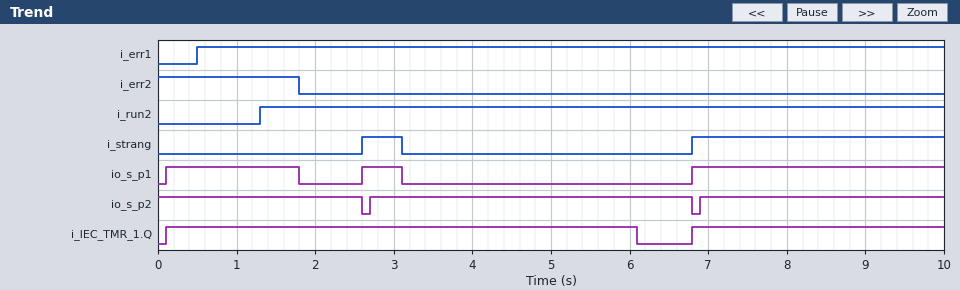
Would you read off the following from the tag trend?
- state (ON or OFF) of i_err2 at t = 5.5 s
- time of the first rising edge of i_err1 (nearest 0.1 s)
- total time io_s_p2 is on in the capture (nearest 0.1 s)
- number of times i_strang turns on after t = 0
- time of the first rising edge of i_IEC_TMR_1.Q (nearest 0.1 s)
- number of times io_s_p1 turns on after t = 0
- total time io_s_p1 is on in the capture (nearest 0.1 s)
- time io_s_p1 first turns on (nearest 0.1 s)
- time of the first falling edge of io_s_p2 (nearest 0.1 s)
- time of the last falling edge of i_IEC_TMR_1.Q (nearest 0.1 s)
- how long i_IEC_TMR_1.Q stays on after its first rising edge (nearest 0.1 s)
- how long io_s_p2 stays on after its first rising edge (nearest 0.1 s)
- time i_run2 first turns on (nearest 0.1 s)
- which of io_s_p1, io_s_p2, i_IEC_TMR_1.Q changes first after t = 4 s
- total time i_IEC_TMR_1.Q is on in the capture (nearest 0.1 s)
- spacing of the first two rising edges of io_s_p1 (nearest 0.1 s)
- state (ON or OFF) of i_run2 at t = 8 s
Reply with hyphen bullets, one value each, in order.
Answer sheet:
- OFF
- 0.5 s
- 9.8 s
- 2
- 0.1 s
- 3
- 5.4 s
- 0.1 s
- 2.6 s
- 6.1 s
- 6.0 s
- 4.1 s
- 1.3 s
- i_IEC_TMR_1.Q
- 9.2 s
- 2.5 s
- ON
